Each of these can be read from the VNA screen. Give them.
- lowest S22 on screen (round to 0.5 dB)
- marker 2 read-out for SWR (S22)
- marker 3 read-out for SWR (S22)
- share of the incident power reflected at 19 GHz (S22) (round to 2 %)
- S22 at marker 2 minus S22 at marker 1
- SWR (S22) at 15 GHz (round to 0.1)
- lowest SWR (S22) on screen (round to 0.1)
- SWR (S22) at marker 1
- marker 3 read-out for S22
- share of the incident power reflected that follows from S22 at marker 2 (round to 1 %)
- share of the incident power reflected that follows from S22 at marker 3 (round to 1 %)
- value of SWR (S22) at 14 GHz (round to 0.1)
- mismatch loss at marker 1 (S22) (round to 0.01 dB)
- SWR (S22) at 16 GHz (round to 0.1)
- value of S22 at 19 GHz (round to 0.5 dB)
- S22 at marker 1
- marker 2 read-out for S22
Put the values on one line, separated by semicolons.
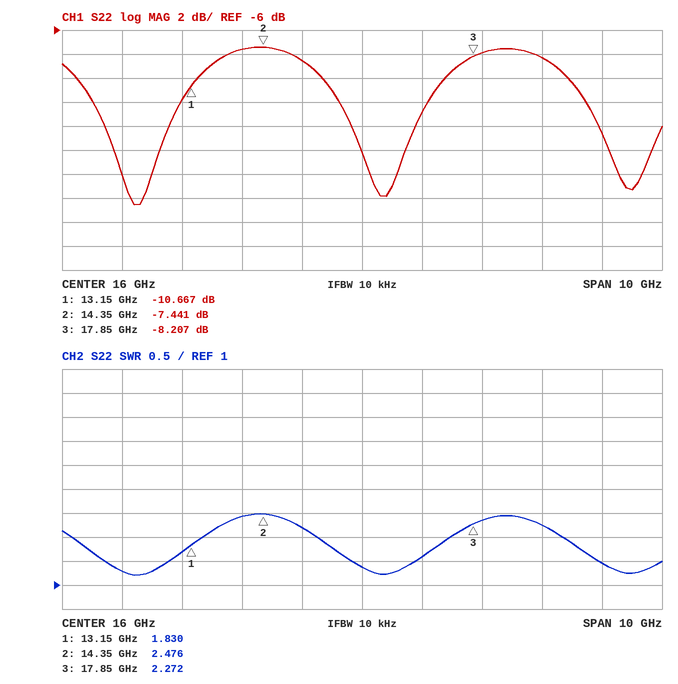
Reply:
-20.5 dB; 2.476; 2.272; 14 %; 3.226 dB; 2.2; 1.2; 1.830; -8.207 dB; 18 %; 15 %; 2.4; 0.39 dB; 1.4; -8.5 dB; -10.667 dB; -7.441 dB
